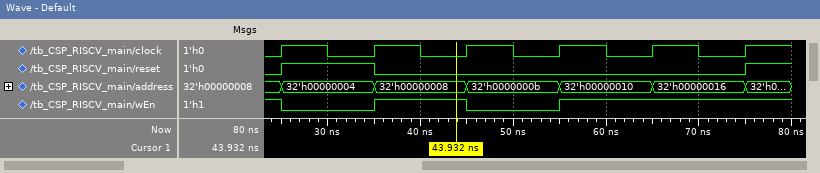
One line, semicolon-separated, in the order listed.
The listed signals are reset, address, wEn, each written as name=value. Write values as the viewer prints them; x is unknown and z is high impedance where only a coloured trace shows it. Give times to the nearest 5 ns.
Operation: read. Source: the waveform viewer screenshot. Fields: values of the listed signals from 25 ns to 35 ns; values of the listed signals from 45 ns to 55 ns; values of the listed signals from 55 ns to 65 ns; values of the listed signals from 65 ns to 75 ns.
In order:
reset=1, address=32'h00000004, wEn=0; reset=0, address=32'h0000000b, wEn=0; reset=0, address=32'h00000010, wEn=1; reset=0, address=32'h00000016, wEn=1
